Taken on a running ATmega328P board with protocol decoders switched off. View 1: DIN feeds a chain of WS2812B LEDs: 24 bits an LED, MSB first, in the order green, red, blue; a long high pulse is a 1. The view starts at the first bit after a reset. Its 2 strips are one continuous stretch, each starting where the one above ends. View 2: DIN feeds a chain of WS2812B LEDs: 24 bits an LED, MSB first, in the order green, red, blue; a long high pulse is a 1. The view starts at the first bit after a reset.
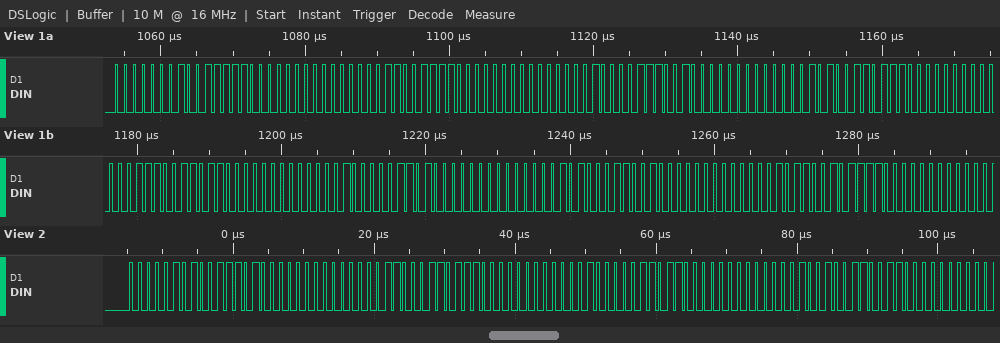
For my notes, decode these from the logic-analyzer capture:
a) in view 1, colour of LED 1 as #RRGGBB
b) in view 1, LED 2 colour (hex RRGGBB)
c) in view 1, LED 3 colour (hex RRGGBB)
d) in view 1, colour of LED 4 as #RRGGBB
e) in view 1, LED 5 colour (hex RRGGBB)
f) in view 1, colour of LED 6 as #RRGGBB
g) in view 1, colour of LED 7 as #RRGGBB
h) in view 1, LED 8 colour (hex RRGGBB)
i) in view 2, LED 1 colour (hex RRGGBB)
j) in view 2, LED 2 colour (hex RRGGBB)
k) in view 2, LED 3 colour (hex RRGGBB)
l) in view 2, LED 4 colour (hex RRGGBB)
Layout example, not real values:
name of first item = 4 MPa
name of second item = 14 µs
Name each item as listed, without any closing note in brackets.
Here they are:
in view 1, colour of LED 1 as #RRGGBB = #3E0100
in view 1, LED 2 colour = #3C0300
in view 1, LED 3 colour = #390400
in view 1, colour of LED 4 as #RRGGBB = #370500
in view 1, LED 5 colour = #360700
in view 1, colour of LED 6 as #RRGGBB = #340800
in view 1, colour of LED 7 as #RRGGBB = #320A00
in view 1, LED 8 colour = #2F0B00
in view 2, LED 1 colour = #3A0500
in view 2, LED 2 colour = #370600
in view 2, LED 3 colour = #360800
in view 2, LED 4 colour = #330900
